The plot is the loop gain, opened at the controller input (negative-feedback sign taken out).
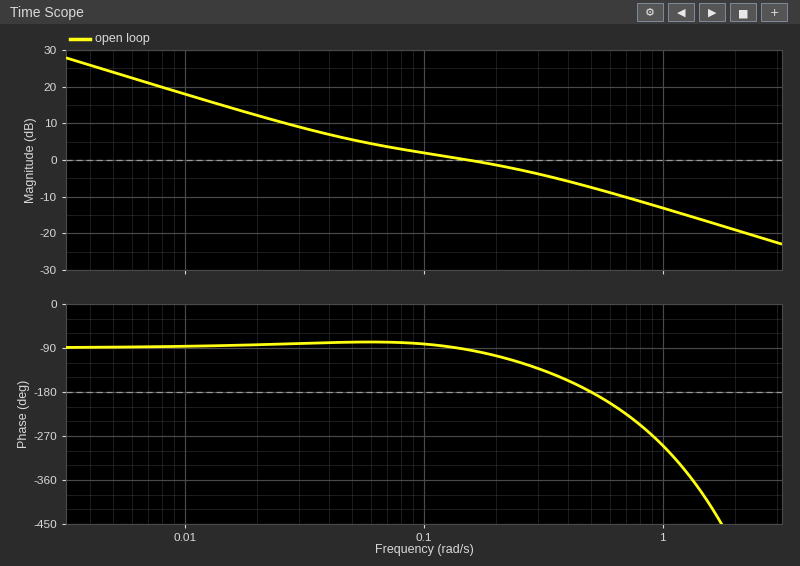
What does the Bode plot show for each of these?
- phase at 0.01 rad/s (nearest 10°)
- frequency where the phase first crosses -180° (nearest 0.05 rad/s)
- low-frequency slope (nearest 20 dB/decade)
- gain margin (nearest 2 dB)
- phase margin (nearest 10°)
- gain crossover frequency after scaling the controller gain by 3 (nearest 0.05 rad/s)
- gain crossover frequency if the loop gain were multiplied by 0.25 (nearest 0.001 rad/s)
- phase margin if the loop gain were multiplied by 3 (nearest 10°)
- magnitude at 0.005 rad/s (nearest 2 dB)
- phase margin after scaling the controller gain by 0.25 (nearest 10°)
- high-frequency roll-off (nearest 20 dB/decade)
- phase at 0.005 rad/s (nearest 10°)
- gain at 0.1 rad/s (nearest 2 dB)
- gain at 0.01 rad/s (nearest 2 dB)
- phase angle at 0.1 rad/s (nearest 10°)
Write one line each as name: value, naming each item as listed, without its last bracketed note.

phase at 0.01 rad/s: -90°
frequency where the phase first crosses -180°: 0.50 rad/s
low-frequency slope: -20 dB/decade
gain margin: 8 dB
phase margin: 90°
gain crossover frequency after scaling the controller gain by 3: 0.65 rad/s
gain crossover frequency if the loop gain were multiplied by 0.25: 0.020 rad/s
phase margin if the loop gain were multiplied by 3: -30°
magnitude at 0.005 rad/s: 24 dB
phase margin after scaling the controller gain by 0.25: 100°
high-frequency roll-off: -20 dB/decade
phase at 0.005 rad/s: -90°
gain at 0.1 rad/s: 2 dB
gain at 0.01 rad/s: 18 dB
phase angle at 0.1 rad/s: -80°
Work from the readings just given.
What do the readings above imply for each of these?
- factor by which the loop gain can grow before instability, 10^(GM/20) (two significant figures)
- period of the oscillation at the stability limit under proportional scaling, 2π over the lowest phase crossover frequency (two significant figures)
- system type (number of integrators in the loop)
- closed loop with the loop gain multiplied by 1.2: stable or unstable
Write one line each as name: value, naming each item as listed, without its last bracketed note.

factor by which the loop gain can grow before instability, 10^(GM/20): 2.5
period of the oscillation at the stability limit under proportional scaling, 2π over the lowest phase crossover frequency: 13 s
system type: 1
closed loop with the loop gain multiplied by 1.2: stable or unstable: stable
